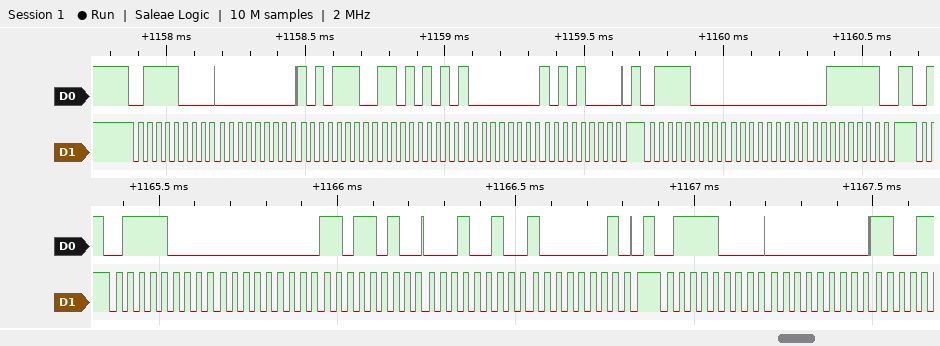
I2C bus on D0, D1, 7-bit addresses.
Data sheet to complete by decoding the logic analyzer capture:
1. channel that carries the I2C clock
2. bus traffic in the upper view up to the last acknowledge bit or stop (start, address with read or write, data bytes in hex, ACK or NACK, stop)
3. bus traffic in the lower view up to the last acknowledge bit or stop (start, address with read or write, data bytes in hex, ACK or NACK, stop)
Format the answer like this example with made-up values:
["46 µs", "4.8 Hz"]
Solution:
["D1", "start, address 3C write ACK, 00 ACK, AE ACK, D5 ACK, 80 ACK, A8 ACK, stop, start, address 3C write ACK, 00 ACK, 3F ACK, stop", "start, address 3C write ACK, 00 ACK, DA ACK, 12 ACK, 81 ACK, stop, start, address 3C write ACK, 00 ACK"]
